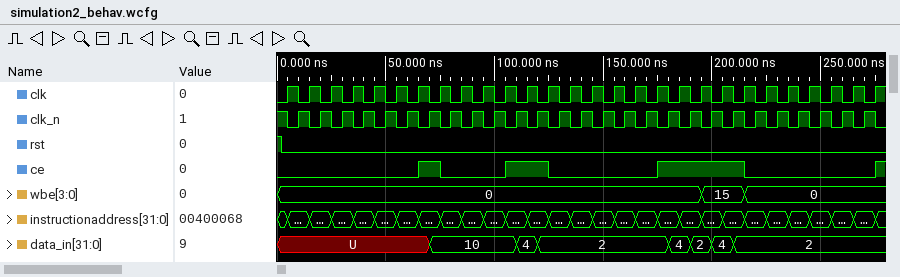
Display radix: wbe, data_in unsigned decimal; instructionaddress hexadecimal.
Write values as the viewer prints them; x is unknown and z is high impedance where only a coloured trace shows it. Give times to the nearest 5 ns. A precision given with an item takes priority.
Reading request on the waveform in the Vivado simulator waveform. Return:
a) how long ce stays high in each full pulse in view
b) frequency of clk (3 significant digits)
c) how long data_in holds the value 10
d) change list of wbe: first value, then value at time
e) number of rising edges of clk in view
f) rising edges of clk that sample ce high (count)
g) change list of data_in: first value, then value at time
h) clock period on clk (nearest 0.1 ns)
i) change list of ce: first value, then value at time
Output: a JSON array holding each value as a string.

["10 ns, 20 ns, 40 ns", "100 MHz", "40 ns", "0, 15 at 195 ns, 0 at 215 ns", "28", "7", "U, 10 at 70 ns, 4 at 110 ns, 2 at 120 ns, 4 at 180 ns, 2 at 190 ns, 4 at 200 ns, 2 at 210 ns", "10 ns", "0, 1 at 65 ns, 0 at 75 ns, 1 at 105 ns, 0 at 125 ns, 1 at 175 ns, 0 at 215 ns, 1 at 275 ns"]
